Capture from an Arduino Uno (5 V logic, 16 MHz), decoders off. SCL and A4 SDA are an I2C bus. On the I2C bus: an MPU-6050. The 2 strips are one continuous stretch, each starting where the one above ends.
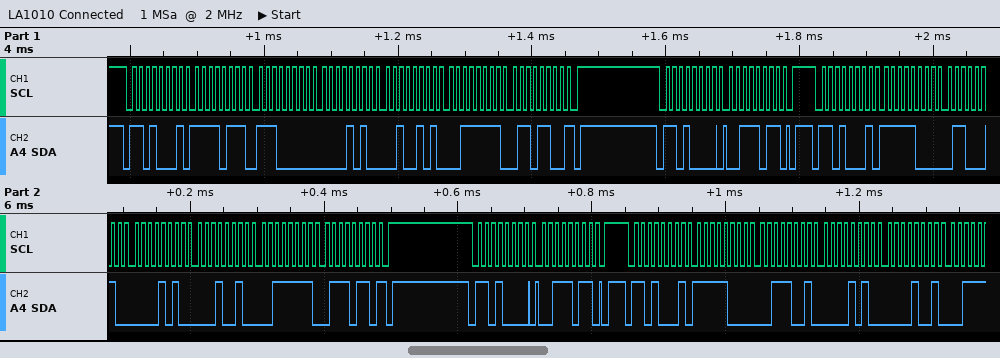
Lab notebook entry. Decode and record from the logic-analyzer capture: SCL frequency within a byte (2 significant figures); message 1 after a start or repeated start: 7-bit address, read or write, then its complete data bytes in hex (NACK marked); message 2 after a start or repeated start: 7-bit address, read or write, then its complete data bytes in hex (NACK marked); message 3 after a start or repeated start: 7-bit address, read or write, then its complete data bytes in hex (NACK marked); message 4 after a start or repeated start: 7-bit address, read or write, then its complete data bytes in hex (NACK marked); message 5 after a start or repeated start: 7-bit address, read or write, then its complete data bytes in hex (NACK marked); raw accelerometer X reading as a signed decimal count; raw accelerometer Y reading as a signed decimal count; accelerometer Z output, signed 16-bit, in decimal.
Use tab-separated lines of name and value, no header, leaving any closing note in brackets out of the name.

SCL frequency within a byte	100 kHz
message 1 after a start or repeated start: 7-bit address, read or write, then its complete data bytes in hex	0x68 read: F7 E0 0A 25 3F 6C NACK
message 2 after a start or repeated start: 7-bit address, read or write, then its complete data bytes in hex	0x68 write: 3B
message 3 after a start or repeated start: 7-bit address, read or write, then its complete data bytes in hex	0x68 read: F8 62 0A 12 3F 76 NACK
message 4 after a start or repeated start: 7-bit address, read or write, then its complete data bytes in hex	0x68 write: 3B
message 5 after a start or repeated start: 7-bit address, read or write, then its complete data bytes in hex	0x68 read: F8 39 0A 09
raw accelerometer X reading as a signed decimal count	-1950
raw accelerometer Y reading as a signed decimal count	2578
accelerometer Z output, signed 16-bit, in decimal	16246
